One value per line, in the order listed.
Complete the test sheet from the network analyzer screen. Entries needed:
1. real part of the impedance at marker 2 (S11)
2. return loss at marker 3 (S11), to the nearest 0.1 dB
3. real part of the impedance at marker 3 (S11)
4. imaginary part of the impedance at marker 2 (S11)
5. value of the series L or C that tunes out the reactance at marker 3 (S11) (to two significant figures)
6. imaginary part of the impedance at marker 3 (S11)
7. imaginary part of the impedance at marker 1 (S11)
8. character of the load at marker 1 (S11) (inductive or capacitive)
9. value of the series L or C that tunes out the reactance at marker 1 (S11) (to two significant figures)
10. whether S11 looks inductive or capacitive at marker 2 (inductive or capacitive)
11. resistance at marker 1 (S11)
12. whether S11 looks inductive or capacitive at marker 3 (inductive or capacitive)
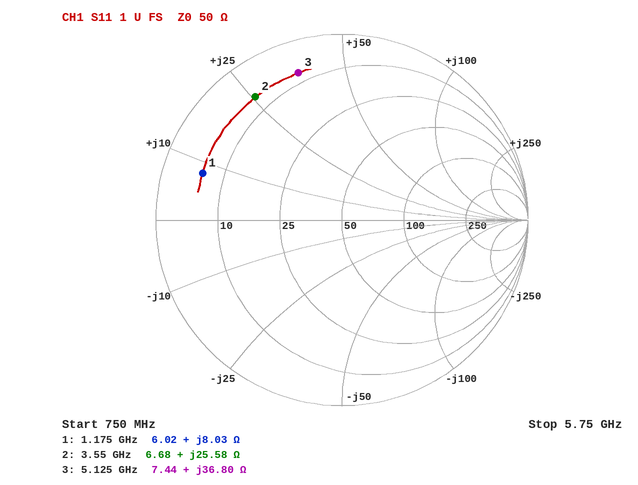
6.68 Ω
1.7 dB
7.44 Ω
+25.58 Ω
840 fF
+36.80 Ω
+8.03 Ω
inductive
17 pF
inductive
6.02 Ω
inductive
